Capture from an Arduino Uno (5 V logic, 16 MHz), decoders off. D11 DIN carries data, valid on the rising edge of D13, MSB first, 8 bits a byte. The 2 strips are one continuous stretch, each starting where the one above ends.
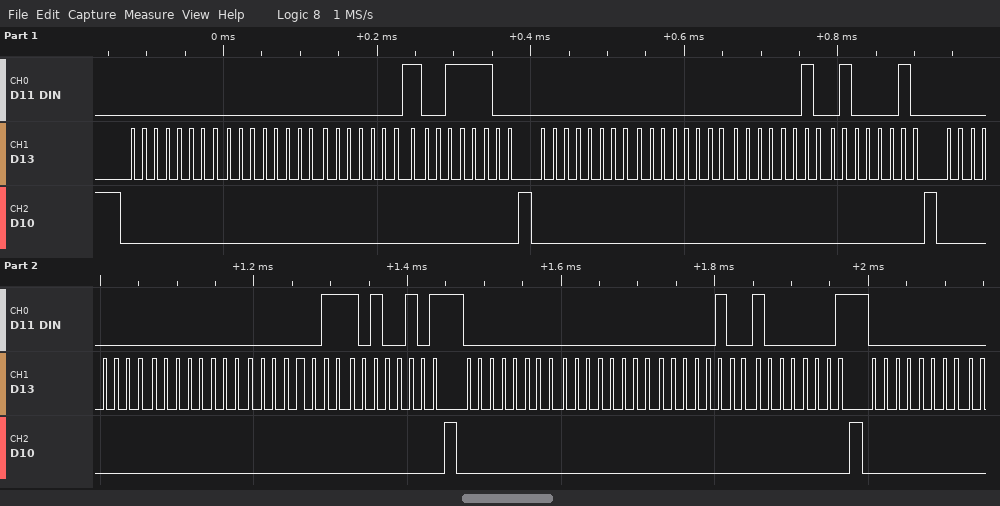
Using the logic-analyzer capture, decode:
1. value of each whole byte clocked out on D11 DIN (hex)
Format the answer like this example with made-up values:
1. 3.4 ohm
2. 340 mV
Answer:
1. 00 00 01 3C 00 00 02 42 00 00 03 A5 00 00 04 81 00
